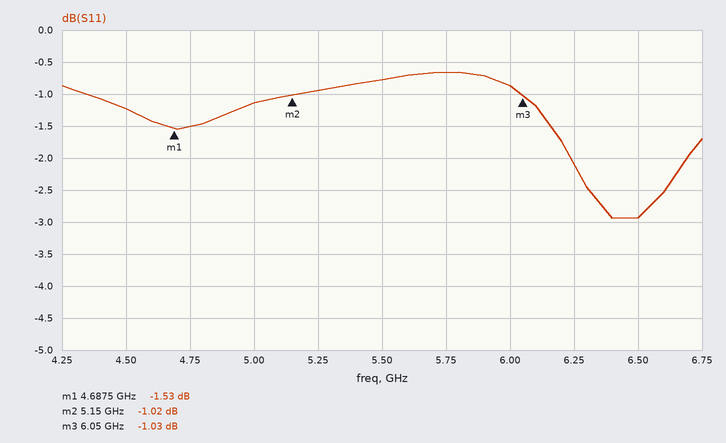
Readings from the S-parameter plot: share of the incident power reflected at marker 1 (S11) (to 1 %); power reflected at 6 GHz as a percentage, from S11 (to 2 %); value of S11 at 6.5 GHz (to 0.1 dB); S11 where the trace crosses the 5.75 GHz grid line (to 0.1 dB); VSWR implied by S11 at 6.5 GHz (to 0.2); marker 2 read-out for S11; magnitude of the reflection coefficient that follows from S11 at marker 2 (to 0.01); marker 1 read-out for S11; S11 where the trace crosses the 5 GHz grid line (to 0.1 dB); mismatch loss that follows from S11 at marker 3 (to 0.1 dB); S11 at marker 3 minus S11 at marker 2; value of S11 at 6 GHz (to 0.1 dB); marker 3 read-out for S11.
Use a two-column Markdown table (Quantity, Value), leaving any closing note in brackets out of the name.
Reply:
| Quantity | Value |
|---|---|
| share of the incident power reflected at marker 1 (S11) | 70 % |
| power reflected at 6 GHz as a percentage, from S11 | 82 % |
| value of S11 at 6.5 GHz | -2.9 dB |
| S11 where the trace crosses the 5.75 GHz grid line | -0.7 dB |
| VSWR implied by S11 at 6.5 GHz | 6.0 |
| marker 2 read-out for S11 | -1.02 dB |
| magnitude of the reflection coefficient that follows from S11 at marker 2 | 0.89 |
| marker 1 read-out for S11 | -1.53 dB |
| S11 where the trace crosses the 5 GHz grid line | -1.1 dB |
| mismatch loss that follows from S11 at marker 3 | 6.8 dB |
| S11 at marker 3 minus S11 at marker 2 | -0.01 dB |
| value of S11 at 6 GHz | -0.9 dB |
| marker 3 read-out for S11 | -1.03 dB |
